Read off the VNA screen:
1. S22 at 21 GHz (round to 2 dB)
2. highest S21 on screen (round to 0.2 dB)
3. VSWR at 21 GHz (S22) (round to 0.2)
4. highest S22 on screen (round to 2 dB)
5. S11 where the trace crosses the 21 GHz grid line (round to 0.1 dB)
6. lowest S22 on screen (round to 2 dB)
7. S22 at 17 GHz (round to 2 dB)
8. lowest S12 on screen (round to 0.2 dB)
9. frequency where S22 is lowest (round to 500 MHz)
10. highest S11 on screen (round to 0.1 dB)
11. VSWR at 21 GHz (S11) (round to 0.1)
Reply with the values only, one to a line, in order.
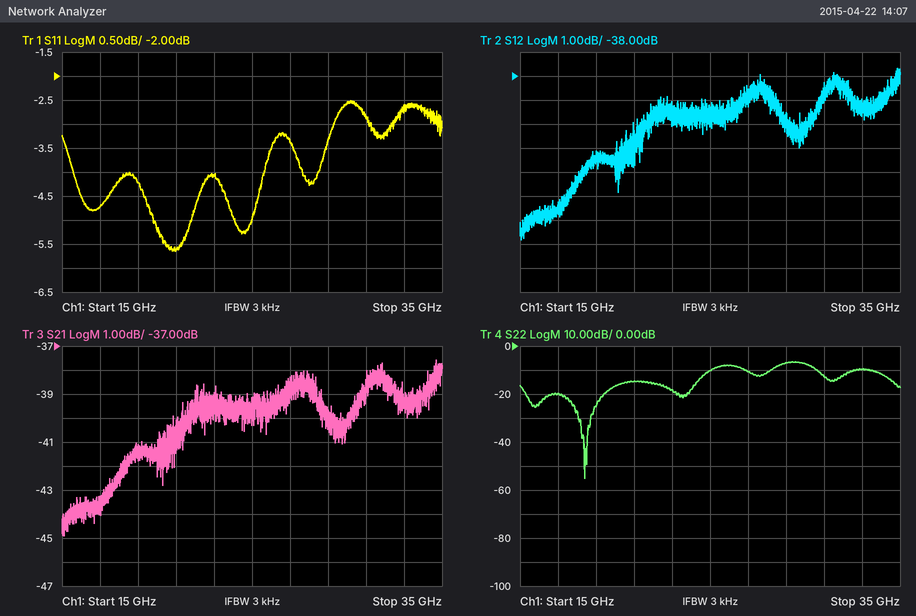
-14 dB
-37.6 dB
1.4
-6 dB
-5.6 dB
-56 dB
-20 dB
-44.8 dB
18.5 GHz
-2.5 dB
3.2
